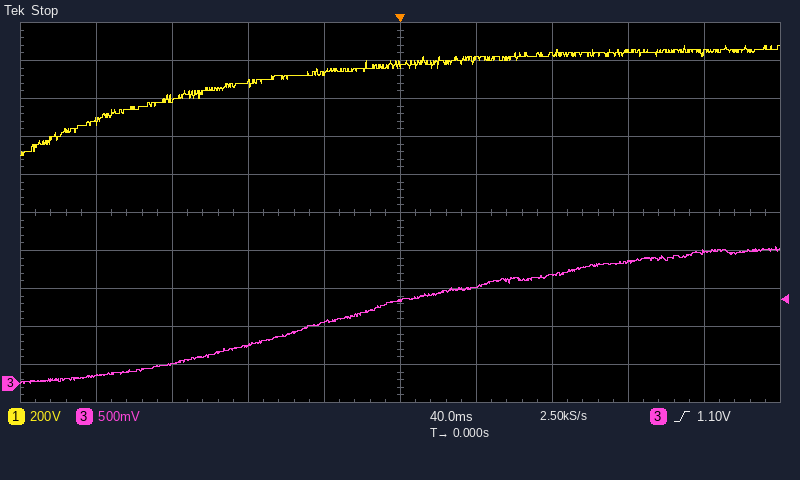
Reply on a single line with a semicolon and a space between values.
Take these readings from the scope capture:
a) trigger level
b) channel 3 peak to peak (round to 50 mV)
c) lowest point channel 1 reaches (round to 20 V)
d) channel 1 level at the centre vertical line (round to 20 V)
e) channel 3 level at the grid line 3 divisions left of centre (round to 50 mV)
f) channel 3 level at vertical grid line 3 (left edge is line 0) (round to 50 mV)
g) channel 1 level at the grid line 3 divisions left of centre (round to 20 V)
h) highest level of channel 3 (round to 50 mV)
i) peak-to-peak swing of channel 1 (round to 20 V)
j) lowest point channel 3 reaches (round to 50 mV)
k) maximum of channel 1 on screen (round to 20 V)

1.10 V; 1.80 V; 1.20 kV; 1.68 kV; 250 mV; 500 mV; 1.50 kV; 1.80 V; 580 V; 0 mV; 1.78 kV
